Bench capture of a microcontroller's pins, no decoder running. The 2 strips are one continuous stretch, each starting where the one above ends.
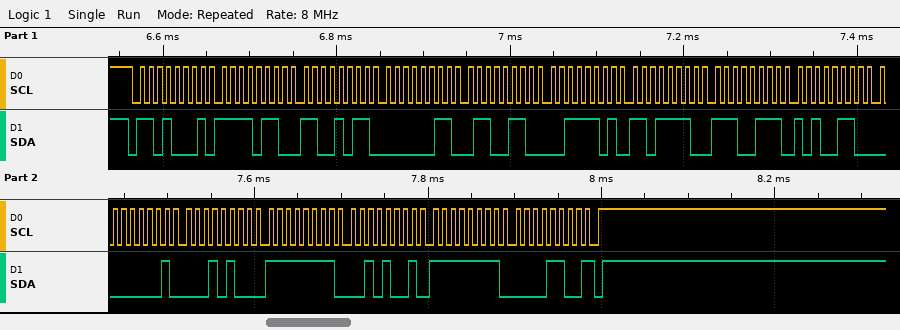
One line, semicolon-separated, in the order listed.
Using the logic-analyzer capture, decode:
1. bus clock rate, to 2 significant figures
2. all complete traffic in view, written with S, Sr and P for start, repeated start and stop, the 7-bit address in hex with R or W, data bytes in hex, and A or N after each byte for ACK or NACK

100 kHz; S 68R A F6 A CB A 03 A 66 A 3D A DE A E7 A A6 A 01 A 14 A FF A 29 A FF A 0C N P
